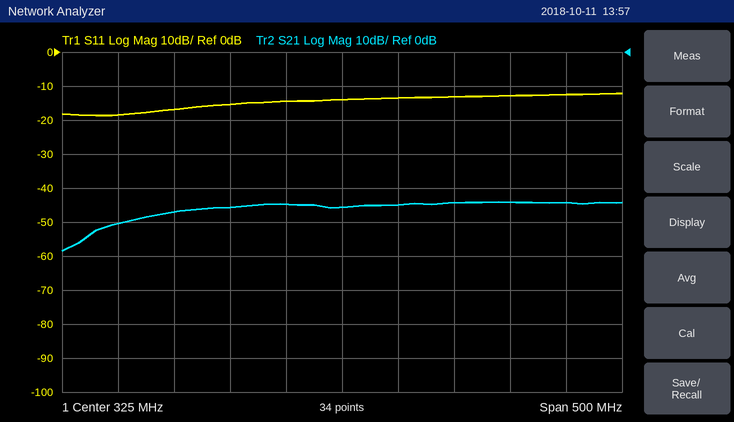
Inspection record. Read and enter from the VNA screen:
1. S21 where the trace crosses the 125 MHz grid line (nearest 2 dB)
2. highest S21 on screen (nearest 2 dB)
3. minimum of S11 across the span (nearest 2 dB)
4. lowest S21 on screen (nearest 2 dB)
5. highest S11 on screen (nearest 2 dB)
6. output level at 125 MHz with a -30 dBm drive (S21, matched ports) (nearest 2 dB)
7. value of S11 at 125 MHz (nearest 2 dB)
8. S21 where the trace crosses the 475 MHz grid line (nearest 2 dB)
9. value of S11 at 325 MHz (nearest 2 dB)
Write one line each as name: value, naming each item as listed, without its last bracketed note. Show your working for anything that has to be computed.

S21 where the trace crosses the 125 MHz grid line: -50 dB
highest S21 on screen: -44 dB
minimum of S11 across the span: -18 dB
lowest S21 on screen: -58 dB
highest S11 on screen: -12 dB
output level at 125 MHz with a -30 dBm drive (S21, matched ports): -30 dBm + (-50 dB) = -80 dBm
value of S11 at 125 MHz: -18 dB
S21 where the trace crosses the 475 MHz grid line: -44 dB
value of S11 at 325 MHz: -14 dB
